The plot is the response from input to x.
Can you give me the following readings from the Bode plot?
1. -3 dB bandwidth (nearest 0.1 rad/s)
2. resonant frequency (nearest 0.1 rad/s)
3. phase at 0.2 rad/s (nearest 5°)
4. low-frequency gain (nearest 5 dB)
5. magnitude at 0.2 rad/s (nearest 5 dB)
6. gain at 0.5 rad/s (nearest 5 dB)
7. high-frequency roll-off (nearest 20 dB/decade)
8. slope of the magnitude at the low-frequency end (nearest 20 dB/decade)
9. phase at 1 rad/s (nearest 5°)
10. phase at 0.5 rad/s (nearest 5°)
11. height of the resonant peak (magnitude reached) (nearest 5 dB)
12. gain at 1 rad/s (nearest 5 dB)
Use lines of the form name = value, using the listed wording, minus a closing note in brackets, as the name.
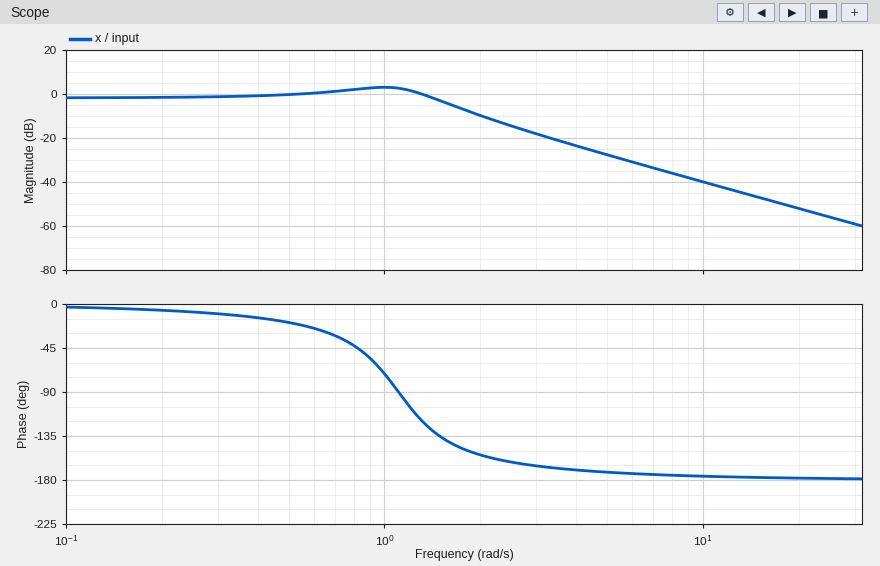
-3 dB bandwidth = 1.6 rad/s
resonant frequency = 1.0 rad/s
phase at 0.2 rad/s = -5°
low-frequency gain = 0 dB
magnitude at 0.2 rad/s = 0 dB
gain at 0.5 rad/s = 0 dB
high-frequency roll-off = -40 dB/decade
slope of the magnitude at the low-frequency end = 0 dB/decade
phase at 1 rad/s = -70°
phase at 0.5 rad/s = -20°
height of the resonant peak (magnitude reached) = 5 dB
gain at 1 rad/s = 5 dB
